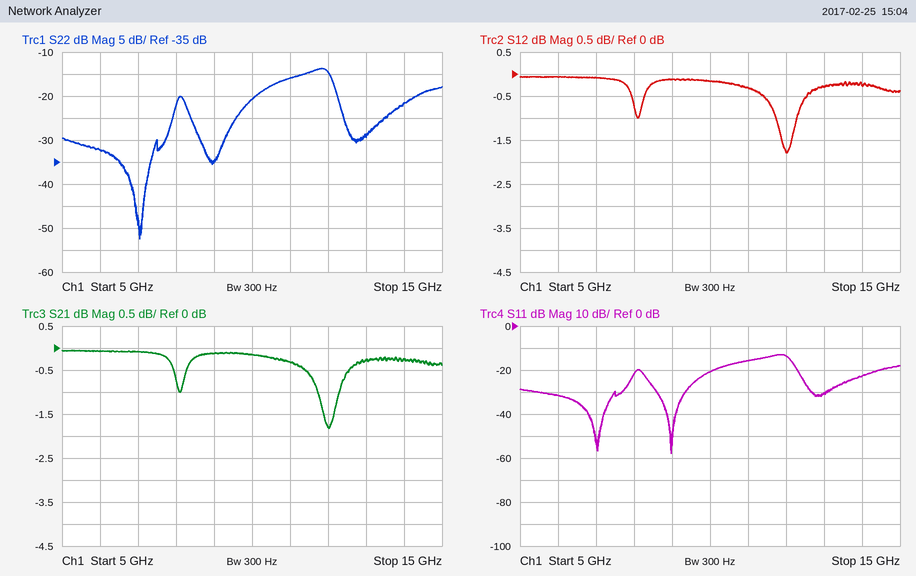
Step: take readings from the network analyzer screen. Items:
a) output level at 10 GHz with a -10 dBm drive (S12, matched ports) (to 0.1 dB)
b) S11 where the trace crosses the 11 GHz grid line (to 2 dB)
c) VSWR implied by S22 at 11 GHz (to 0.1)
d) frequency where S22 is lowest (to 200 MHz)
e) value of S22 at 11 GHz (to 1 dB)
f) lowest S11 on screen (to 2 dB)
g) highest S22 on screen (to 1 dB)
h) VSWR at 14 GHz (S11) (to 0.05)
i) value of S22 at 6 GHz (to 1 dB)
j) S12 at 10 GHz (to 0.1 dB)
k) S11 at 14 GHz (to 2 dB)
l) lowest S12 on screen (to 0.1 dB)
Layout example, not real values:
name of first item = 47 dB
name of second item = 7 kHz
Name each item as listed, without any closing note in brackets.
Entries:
output level at 10 GHz with a -10 dBm drive (S12, matched ports) = -10.2 dBm
S11 where the trace crosses the 11 GHz grid line = -16 dB
VSWR implied by S22 at 11 GHz = 1.4
frequency where S22 is lowest = 7.0 GHz
value of S22 at 11 GHz = -16 dB
lowest S11 on screen = -58 dB
highest S22 on screen = -14 dB
VSWR at 14 GHz (S11) = 1.15
value of S22 at 6 GHz = -32 dB
S12 at 10 GHz = -0.2 dB
S11 at 14 GHz = -22 dB
lowest S12 on screen = -1.8 dB
